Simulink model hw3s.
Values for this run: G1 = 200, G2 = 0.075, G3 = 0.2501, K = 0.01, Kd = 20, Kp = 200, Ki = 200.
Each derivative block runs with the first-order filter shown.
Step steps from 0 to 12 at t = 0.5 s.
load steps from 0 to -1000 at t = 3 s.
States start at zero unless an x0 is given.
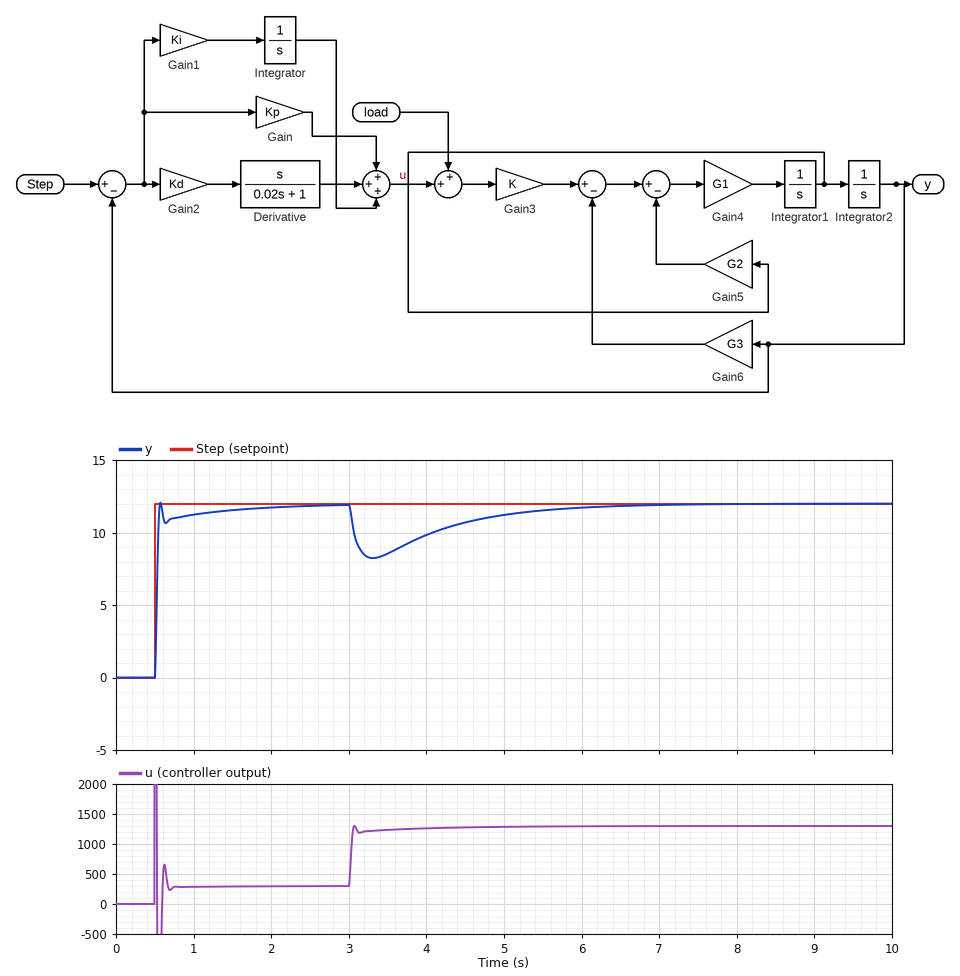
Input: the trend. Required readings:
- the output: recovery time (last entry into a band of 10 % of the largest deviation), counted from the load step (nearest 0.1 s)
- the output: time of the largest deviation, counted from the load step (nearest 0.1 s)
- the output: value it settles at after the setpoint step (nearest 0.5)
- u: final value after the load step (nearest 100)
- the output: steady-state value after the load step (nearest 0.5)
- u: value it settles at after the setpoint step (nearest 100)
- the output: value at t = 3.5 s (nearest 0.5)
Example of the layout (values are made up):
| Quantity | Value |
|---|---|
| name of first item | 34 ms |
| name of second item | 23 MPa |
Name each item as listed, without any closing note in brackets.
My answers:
| Quantity | Value |
|---|---|
| the output: recovery time (last entry into a band of 10 % of the largest deviation), counted from the load step | 2.8 s |
| the output: time of the largest deviation, counted from the load step | 0.3 s |
| the output: value it settles at after the setpoint step | 12.0 |
| u: final value after the load step | 1300 |
| the output: steady-state value after the load step | 12.0 |
| u: value it settles at after the setpoint step | 300 |
| the output: value at t = 3.5 s | 8.5 |
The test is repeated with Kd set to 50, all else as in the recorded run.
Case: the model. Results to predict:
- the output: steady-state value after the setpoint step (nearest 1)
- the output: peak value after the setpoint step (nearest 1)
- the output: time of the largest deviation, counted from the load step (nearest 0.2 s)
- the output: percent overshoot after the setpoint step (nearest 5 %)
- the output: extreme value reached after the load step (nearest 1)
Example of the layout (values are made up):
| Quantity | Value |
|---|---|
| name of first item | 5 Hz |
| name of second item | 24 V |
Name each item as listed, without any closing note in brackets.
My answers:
| Quantity | Value |
|---|---|
| the output: steady-state value after the setpoint step | 12 |
| the output: peak value after the setpoint step | 14 |
| the output: time of the largest deviation, counted from the load step | 0.6 s |
| the output: percent overshoot after the setpoint step | 15 % |
| the output: extreme value reached after the load step | 9 |
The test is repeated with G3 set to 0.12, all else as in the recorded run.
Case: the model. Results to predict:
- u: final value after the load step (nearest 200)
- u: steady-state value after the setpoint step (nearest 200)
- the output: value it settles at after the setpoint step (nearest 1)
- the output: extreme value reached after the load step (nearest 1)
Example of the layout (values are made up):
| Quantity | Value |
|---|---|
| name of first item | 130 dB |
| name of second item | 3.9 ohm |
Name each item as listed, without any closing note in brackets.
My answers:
| Quantity | Value |
|---|---|
| u: final value after the load step | 1200 |
| u: steady-state value after the setpoint step | 200 |
| the output: value it settles at after the setpoint step | 12 |
| the output: extreme value reached after the load step | 8 |
